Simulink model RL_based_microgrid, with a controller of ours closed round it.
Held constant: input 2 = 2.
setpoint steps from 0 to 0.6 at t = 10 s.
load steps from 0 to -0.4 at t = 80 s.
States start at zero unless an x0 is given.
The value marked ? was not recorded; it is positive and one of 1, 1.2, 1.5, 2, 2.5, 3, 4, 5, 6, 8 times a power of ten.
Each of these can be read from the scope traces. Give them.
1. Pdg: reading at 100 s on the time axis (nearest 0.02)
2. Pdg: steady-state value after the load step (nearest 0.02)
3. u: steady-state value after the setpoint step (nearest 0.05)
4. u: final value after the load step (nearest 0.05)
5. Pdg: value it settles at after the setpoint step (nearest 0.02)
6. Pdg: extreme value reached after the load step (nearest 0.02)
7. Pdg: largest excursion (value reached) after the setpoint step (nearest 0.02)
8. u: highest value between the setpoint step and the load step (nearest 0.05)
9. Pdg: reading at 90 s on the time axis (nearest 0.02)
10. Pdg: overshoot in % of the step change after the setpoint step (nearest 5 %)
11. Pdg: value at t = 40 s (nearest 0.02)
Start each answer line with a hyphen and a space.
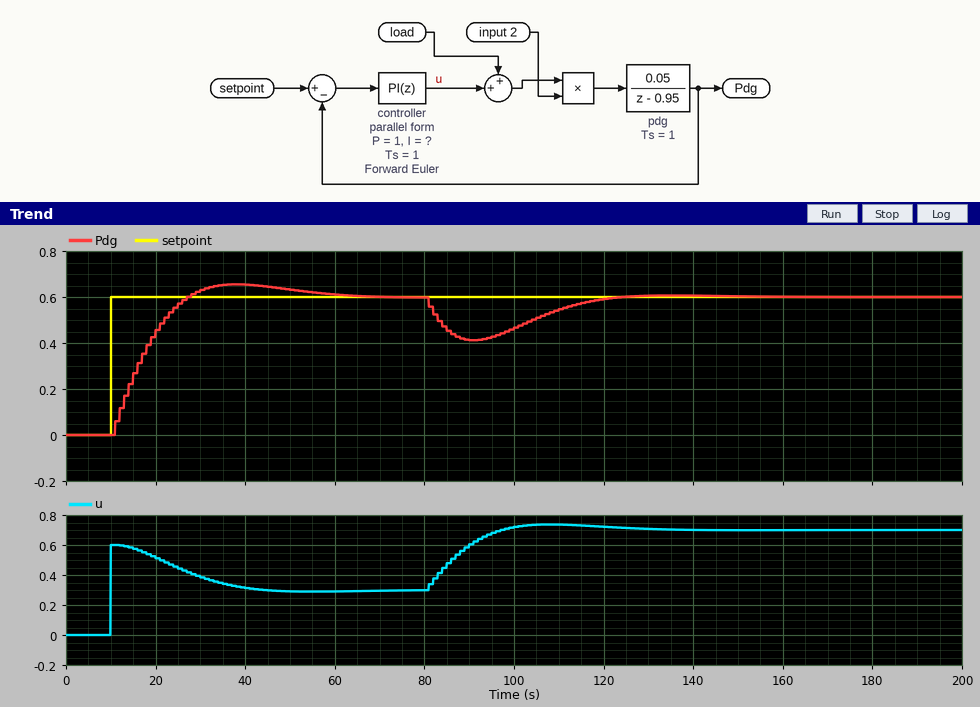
- 0.46
- 0.60
- 0.30
- 0.70
- 0.60
- 0.42
- 0.66
- 0.60
- 0.42
- 10 %
- 0.66
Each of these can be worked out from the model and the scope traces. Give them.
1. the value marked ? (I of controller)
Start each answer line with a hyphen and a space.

- 0.1
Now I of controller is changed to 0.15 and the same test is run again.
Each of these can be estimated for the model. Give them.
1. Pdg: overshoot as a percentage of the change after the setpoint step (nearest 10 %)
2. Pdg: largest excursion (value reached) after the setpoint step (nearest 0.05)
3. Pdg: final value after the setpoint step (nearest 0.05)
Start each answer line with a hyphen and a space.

- 20 %
- 0.70
- 0.60
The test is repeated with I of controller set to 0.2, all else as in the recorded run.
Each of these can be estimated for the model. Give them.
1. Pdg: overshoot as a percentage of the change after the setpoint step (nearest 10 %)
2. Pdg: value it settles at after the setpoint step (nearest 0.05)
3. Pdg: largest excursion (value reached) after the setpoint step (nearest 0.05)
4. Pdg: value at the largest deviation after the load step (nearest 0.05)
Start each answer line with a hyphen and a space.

- 20 %
- 0.60
- 0.75
- 0.45
